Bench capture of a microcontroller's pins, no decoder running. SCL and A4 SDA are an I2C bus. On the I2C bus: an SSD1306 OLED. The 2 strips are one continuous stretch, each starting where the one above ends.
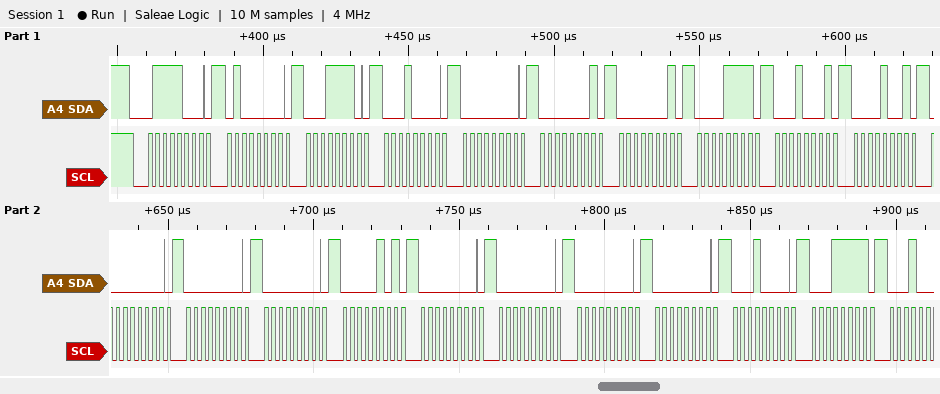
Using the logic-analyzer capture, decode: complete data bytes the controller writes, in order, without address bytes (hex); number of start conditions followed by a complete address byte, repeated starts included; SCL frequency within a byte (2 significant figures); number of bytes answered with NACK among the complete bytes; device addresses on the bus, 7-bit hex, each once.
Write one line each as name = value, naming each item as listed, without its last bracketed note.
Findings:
complete data bytes the controller writes, in order, without address bytes = 40 1E 10 00 01 01 0F 11 09 00 00 00 05 00 00 00 00 10 1F
number of start conditions followed by a complete address byte, repeated starts included = 1
SCL frequency within a byte = 400 kHz
number of bytes answered with NACK among the complete bytes = 0
device addresses on the bus, 7-bit hex, each once = 0x3C
